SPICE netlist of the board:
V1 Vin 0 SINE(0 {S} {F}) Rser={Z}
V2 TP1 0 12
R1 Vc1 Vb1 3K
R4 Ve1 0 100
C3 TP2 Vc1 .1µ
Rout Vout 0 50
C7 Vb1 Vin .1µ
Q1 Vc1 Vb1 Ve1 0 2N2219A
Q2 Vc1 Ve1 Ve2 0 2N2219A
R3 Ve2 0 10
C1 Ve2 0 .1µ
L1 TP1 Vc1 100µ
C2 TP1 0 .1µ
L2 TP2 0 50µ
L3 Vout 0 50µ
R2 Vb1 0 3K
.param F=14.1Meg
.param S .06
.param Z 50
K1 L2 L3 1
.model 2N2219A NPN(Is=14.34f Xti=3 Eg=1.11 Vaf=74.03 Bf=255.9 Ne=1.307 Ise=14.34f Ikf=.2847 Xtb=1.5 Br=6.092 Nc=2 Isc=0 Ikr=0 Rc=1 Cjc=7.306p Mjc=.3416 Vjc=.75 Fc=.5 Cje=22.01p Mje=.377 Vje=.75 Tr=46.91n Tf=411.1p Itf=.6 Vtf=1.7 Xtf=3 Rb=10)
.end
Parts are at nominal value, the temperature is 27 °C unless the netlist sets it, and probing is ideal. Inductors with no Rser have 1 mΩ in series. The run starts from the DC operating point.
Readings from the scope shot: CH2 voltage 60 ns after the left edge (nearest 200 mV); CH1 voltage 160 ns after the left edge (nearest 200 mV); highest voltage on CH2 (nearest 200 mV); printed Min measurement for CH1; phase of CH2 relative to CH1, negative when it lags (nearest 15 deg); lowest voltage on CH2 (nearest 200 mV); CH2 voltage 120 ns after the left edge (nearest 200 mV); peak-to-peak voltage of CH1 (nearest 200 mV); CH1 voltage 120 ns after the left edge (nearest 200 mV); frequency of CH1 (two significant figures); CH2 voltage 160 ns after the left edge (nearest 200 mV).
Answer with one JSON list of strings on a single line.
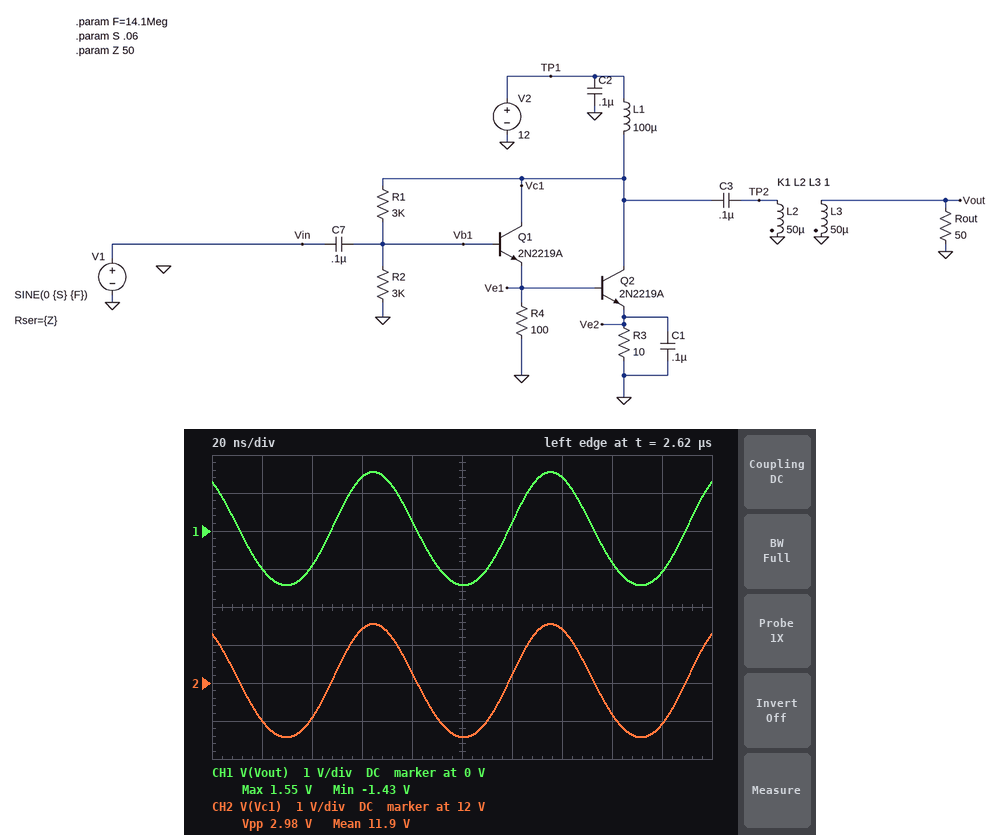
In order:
["13.4 V", "-800 mV", "13.6 V", "-1.43 V", "0 deg", "10.6 V", "12.2 V", "3.0 V", "200 mV", "14 MHz", "11.2 V"]
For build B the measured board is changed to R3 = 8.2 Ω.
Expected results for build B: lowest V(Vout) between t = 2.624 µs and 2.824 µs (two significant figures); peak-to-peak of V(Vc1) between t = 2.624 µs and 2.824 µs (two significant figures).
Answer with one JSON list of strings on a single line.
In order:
["-1.3 V", "2.8 V"]
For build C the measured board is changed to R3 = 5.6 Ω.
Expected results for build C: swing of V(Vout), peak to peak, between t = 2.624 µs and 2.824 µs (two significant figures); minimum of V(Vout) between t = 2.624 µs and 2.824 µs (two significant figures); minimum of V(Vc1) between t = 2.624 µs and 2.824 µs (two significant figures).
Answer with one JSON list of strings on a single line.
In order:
["2.4 V", "-1.1 V", "11 V"]
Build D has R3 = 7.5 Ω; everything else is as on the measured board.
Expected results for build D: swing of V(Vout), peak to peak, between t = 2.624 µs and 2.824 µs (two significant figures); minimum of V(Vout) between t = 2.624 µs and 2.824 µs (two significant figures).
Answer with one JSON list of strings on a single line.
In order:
["2.7 V", "-1.3 V"]
